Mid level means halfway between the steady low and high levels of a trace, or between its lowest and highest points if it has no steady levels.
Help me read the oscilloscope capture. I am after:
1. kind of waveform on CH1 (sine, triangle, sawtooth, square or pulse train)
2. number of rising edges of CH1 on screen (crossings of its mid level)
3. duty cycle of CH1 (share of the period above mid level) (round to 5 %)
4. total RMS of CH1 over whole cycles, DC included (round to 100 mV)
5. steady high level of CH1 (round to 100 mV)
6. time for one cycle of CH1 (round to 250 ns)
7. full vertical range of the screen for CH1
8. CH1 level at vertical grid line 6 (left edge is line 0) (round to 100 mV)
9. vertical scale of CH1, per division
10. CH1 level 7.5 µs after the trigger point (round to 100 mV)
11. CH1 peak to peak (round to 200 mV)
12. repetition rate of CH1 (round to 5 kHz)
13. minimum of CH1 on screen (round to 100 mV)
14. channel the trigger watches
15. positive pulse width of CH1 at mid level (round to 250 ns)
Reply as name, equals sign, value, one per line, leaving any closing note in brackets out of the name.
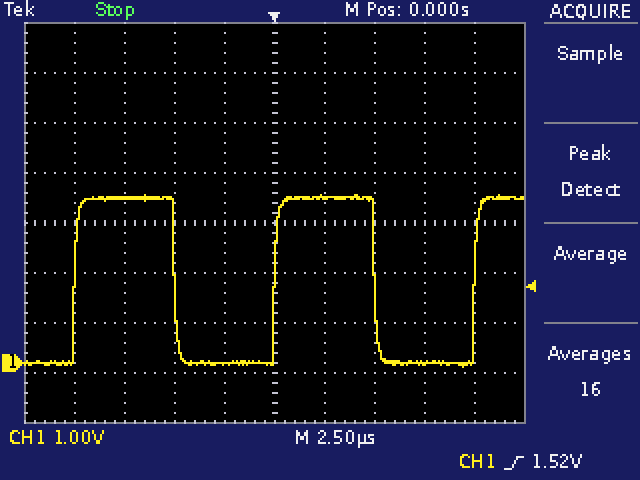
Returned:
kind of waveform on CH1 = square
number of rising edges of CH1 on screen = 3
duty cycle of CH1 (share of the period above mid level) = 50 %
total RMS of CH1 over whole cycles, DC included = 2.3 V
steady high level of CH1 = 3.3 V
time for one cycle of CH1 = 10.00 µs
full vertical range of the screen for CH1 = 8 V
CH1 level at vertical grid line 6 (left edge is line 0) = 3.3 V
vertical scale of CH1, per division = 1 V
CH1 level 7.5 µs after the trigger point = 0.0 V
CH1 peak to peak = 3.4 V
repetition rate of CH1 = 100 kHz
minimum of CH1 on screen = -100 mV
channel the trigger watches = CH1
positive pulse width of CH1 at mid level = 5.00 µs
